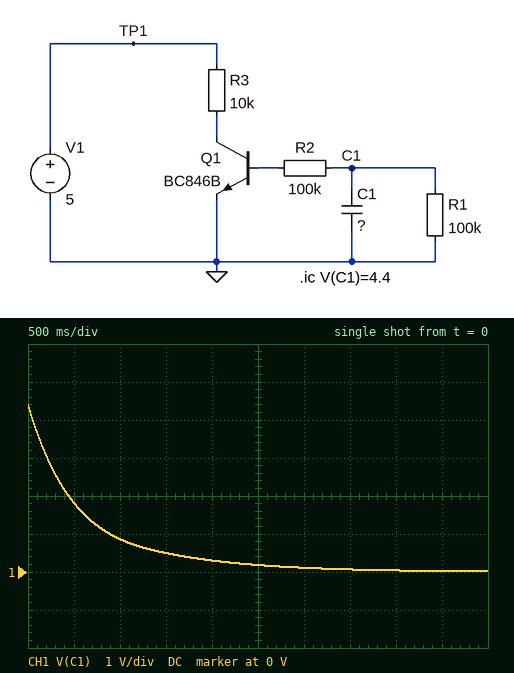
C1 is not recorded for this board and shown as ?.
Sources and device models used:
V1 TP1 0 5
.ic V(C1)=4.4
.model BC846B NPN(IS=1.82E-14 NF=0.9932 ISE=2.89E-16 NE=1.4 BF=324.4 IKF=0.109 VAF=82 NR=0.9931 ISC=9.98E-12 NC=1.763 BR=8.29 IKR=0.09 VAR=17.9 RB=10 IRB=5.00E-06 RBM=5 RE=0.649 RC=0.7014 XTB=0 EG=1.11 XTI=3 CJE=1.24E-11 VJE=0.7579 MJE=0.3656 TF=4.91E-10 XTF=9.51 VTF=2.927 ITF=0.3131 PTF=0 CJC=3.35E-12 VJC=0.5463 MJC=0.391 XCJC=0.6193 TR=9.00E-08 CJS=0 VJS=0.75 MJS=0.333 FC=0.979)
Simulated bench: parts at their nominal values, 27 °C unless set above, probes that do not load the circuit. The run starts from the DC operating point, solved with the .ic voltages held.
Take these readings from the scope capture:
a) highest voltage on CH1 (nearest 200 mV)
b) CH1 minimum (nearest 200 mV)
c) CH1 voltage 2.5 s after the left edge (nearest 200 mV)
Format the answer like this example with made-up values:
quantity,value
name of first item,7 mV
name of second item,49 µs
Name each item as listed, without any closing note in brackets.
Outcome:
quantity,value
highest voltage on CH1,4.4 V
CH1 minimum,0 V
CH1 voltage 2.5 s after the left edge,200 mV
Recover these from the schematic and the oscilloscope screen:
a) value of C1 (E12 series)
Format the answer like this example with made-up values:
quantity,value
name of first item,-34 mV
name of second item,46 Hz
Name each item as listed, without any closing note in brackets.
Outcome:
quantity,value
value of C1,10 µF
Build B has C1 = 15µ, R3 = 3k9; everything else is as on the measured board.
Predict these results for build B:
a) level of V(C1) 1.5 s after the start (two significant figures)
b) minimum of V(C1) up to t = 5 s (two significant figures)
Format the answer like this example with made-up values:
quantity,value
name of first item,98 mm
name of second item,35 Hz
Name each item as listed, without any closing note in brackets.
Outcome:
quantity,value
level of V(C1) 1.5 s after the start,870 mV
minimum of V(C1) up to t = 5 s,80 mV
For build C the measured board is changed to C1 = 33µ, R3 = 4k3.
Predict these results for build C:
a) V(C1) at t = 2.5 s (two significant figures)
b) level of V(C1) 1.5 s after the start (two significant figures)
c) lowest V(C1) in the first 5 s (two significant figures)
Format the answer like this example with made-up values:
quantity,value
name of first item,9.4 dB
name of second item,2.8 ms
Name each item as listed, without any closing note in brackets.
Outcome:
quantity,value
V(C1) at t = 2.5 s,1.2 V
level of V(C1) 1.5 s after the start,2.0 V
lowest V(C1) in the first 5 s,490 mV
